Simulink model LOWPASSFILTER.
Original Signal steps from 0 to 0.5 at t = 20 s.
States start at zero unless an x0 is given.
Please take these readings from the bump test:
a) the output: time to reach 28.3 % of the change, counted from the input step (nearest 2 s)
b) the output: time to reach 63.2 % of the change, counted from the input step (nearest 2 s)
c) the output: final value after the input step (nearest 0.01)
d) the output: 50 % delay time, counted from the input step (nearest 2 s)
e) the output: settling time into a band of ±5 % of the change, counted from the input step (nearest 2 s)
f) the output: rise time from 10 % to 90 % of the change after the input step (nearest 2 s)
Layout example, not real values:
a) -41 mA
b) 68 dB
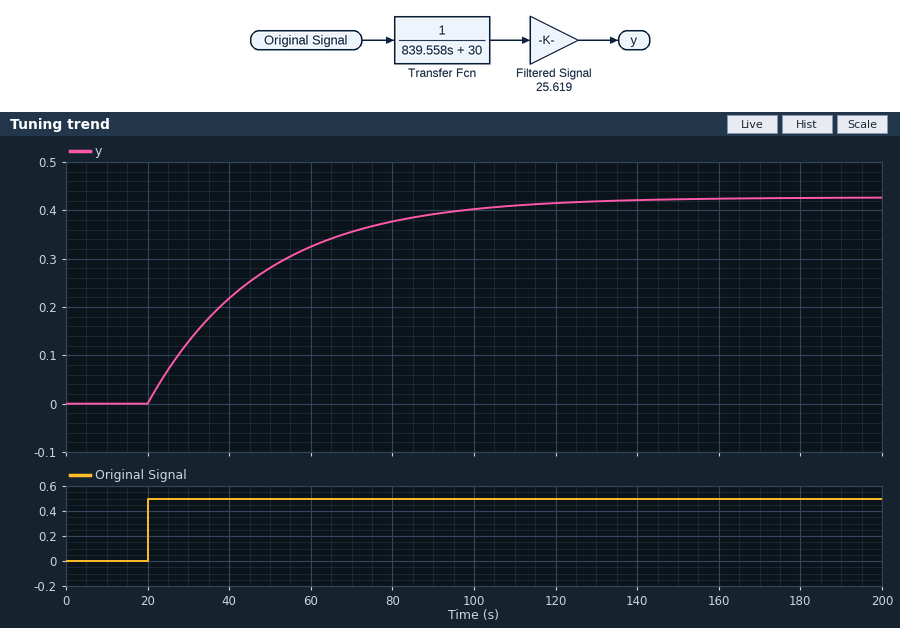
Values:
a) 10 s
b) 28 s
c) 0.43
d) 20 s
e) 84 s
f) 62 s
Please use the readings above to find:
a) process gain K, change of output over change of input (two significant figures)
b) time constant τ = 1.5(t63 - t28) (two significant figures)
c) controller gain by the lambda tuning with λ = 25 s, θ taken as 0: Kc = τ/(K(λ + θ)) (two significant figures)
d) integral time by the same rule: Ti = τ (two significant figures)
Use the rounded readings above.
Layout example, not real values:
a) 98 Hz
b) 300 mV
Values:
a) 0.86
b) 27 s
c) 1.3
d) 27 s
